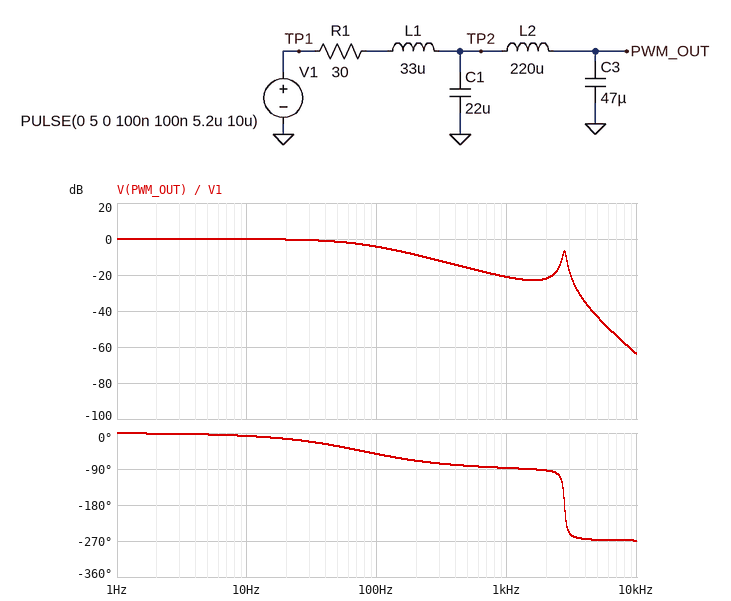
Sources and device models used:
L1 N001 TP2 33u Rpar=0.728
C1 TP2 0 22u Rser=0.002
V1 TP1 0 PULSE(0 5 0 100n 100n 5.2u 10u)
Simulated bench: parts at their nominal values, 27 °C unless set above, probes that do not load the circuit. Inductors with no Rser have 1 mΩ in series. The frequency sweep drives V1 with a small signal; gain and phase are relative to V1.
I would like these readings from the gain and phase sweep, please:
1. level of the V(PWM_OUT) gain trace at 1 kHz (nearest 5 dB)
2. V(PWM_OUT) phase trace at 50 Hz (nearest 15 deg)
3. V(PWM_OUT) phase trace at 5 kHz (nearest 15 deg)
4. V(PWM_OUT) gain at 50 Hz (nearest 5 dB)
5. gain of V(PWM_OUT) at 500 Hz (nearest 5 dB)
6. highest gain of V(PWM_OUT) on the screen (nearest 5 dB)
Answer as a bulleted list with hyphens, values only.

- -20 dB
- -30 deg
- -270 deg
- 0 dB
- -15 dB
- 0 dB
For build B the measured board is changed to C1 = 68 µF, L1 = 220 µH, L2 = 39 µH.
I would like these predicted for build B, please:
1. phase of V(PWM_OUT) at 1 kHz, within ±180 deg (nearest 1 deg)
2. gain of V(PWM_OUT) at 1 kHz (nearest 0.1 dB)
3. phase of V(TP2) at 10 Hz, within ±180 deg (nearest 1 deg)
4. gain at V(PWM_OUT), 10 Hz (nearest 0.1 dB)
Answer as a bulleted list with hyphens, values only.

- -88 deg
- -26.5 dB
- -12 deg
- -0.2 dB
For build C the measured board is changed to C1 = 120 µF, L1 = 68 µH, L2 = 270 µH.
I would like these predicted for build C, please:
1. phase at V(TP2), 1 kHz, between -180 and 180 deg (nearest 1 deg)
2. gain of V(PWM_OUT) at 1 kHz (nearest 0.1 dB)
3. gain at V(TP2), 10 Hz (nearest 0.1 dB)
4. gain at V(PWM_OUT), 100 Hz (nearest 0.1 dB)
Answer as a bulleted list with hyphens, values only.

- -89 deg
- -26.1 dB
- -0.4 dB
- -10.3 dB
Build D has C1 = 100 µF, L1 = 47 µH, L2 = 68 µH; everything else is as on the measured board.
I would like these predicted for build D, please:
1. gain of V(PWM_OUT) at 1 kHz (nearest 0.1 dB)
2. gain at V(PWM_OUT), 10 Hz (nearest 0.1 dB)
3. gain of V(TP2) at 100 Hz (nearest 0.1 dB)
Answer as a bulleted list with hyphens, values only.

- -28.1 dB
- -0.3 dB
- -9.4 dB
